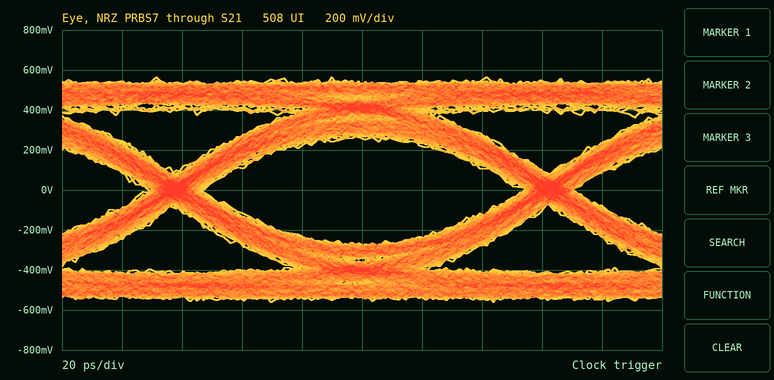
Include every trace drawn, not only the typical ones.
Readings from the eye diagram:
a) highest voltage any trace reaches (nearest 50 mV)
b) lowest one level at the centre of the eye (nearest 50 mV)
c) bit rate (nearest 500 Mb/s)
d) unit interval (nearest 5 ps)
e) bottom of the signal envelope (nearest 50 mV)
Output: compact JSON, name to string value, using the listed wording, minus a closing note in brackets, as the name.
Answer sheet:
{"highest voltage any trace reaches": "550 mV", "lowest one level at the centre of the eye": "250 mV", "bit rate": "8.0 Gb/s", "unit interval": "125 ps", "bottom of the signal envelope": "-550 mV"}
